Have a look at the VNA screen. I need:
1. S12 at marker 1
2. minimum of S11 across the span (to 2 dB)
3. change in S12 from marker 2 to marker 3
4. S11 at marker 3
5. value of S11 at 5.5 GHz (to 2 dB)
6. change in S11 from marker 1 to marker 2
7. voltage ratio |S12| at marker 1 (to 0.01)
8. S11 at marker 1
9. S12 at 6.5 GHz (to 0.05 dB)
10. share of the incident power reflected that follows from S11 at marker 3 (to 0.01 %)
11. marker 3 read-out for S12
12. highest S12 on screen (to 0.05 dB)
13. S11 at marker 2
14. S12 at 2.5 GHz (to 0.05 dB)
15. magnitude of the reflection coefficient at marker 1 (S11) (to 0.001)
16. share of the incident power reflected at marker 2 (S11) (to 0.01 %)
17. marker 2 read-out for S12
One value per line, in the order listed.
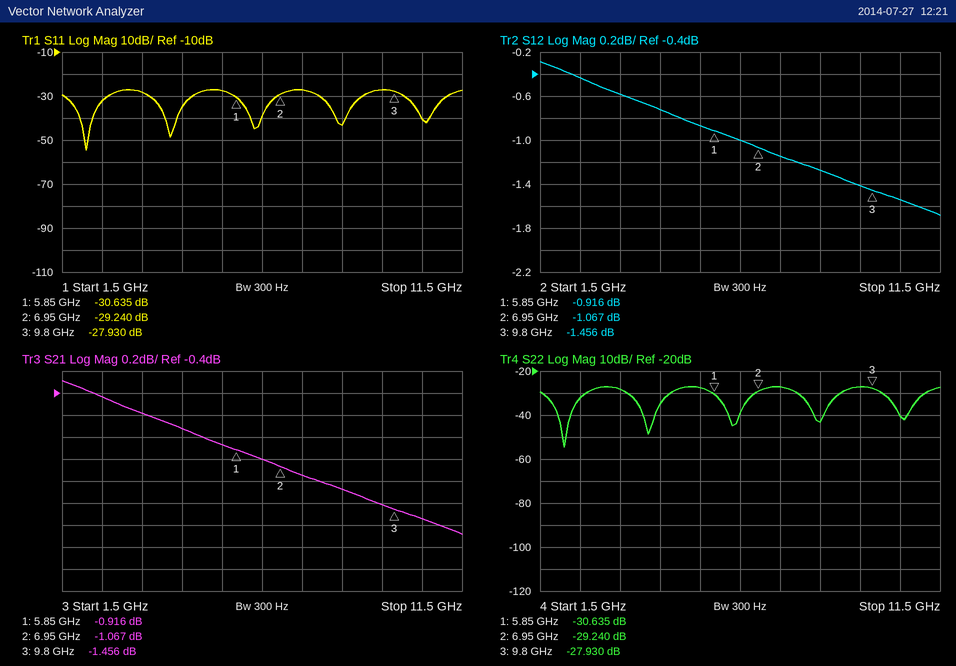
-0.916 dB
-54 dB
-0.389 dB
-27.930 dB
-28 dB
1.395 dB
0.90
-30.635 dB
-1.00 dB
0.16 %
-1.456 dB
-0.30 dB
-29.240 dB
-0.45 dB
0.029
0.12 %
-1.067 dB
